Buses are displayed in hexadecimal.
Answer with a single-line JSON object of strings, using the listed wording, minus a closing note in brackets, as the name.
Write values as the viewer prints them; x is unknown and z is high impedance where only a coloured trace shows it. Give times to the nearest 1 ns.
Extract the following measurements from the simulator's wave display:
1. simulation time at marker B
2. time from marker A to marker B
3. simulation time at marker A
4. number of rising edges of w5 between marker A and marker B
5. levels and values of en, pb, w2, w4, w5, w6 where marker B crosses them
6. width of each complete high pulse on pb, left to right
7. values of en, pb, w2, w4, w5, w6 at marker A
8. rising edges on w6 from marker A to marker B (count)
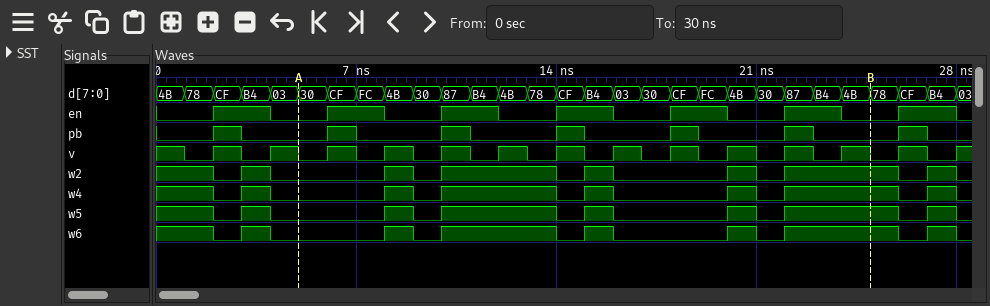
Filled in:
{"simulation time at marker B": "25 ns", "time from marker A to marker B": "20 ns", "simulation time at marker A": "5 ns", "number of rising edges of w5 between marker A and marker B": "5", "levels and values of en, pb, w2, w4, w5, w6 where marker B crosses them": "en=0, pb=0, w2=1, w4=1, w5=1, w6=1", "width of each complete high pulse on pb, left to right": "1 ns, 1 ns, 1 ns, 1 ns, 1 ns, 1 ns, 1 ns", "values of en, pb, w2, w4, w5, w6 at marker A": "en=0, pb=0, w2=0, w4=0, w5=0, w6=0", "rising edges on w6 from marker A to marker B": "5"}
